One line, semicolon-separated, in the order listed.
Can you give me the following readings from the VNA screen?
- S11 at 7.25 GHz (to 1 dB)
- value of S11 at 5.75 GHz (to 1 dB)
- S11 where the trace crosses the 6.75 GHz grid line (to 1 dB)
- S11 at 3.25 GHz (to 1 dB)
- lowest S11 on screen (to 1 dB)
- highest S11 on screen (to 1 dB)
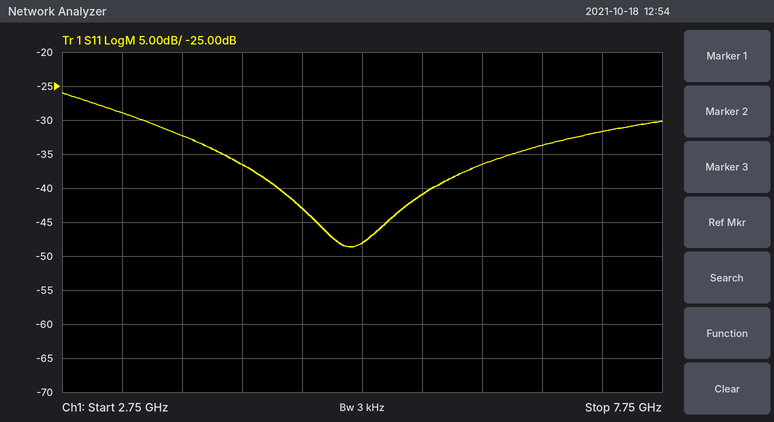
-32 dB; -41 dB; -34 dB; -29 dB; -49 dB; -26 dB
